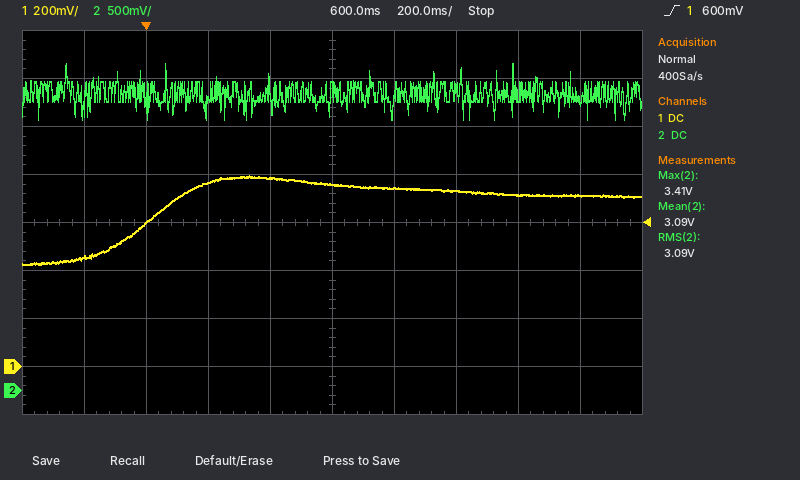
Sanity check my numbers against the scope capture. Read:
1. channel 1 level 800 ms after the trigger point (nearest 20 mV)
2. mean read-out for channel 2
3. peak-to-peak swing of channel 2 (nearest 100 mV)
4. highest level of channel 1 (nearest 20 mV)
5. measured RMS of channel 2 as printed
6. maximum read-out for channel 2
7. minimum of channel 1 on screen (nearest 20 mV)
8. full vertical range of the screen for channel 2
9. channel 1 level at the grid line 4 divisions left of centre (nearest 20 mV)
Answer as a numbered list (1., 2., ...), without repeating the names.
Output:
1. 740 mV
2. 3.09 V
3. 600 mV
4. 800 mV
5. 3.09 V
6. 3.41 V
7. 420 mV
8. 4 V
9. 460 mV
